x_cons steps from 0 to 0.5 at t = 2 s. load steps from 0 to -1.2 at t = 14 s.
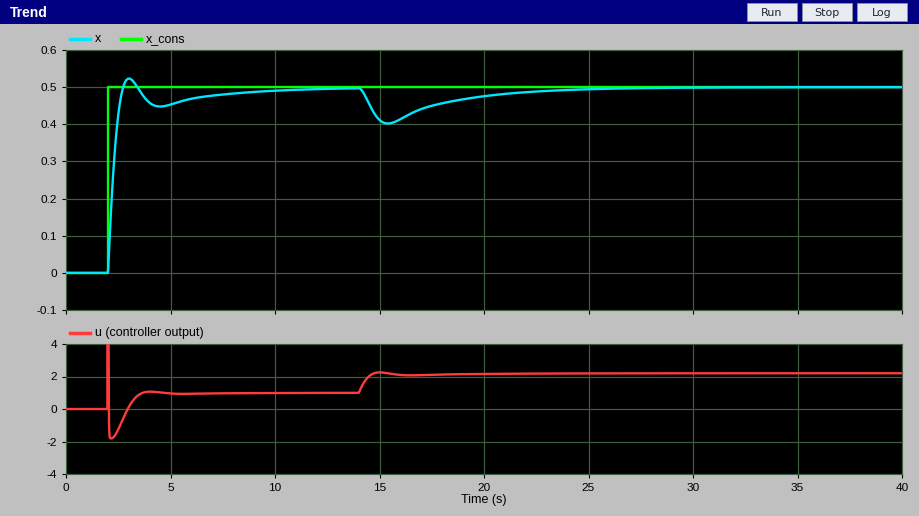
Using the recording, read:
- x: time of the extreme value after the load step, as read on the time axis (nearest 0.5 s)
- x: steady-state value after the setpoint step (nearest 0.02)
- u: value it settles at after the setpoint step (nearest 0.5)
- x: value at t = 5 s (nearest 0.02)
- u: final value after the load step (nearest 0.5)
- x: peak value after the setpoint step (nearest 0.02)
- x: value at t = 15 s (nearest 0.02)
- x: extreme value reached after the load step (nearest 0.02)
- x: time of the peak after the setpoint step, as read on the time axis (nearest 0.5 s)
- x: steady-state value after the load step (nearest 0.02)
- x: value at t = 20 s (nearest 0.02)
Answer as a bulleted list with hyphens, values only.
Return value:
- 15.5 s
- 0.50
- 1.0
- 0.46
- 2.0
- 0.52
- 0.42
- 0.40
- 3.0 s
- 0.50
- 0.48
